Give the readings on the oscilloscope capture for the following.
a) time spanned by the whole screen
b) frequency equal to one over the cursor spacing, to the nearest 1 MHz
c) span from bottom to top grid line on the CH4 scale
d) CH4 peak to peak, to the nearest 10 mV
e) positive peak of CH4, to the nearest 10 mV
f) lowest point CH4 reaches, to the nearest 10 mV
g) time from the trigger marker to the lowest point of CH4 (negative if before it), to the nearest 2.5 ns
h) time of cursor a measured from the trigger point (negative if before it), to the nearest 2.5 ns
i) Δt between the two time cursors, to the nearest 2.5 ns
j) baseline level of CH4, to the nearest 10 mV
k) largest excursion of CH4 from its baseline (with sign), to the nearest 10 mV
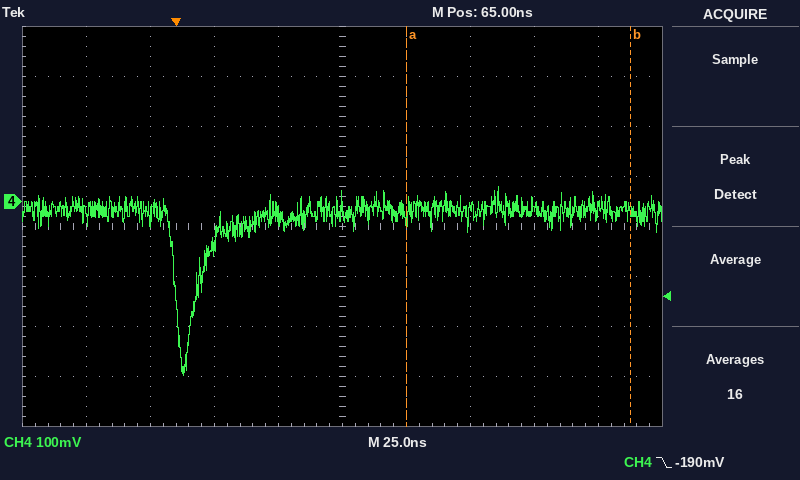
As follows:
250 ns
11 MHz
800 mV
380 mV
30 mV
-350 mV
+2.5 ns
+90.0 ns
87.5 ns
-20 mV
-330 mV
